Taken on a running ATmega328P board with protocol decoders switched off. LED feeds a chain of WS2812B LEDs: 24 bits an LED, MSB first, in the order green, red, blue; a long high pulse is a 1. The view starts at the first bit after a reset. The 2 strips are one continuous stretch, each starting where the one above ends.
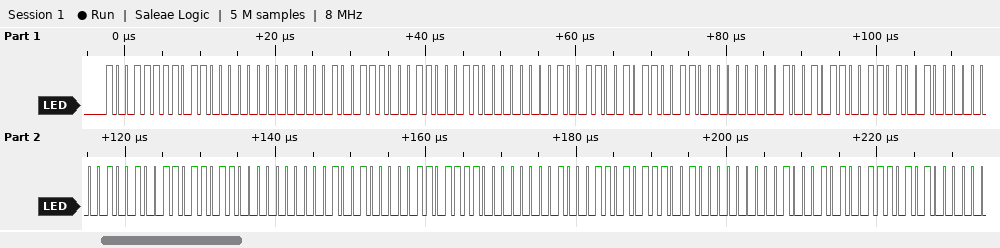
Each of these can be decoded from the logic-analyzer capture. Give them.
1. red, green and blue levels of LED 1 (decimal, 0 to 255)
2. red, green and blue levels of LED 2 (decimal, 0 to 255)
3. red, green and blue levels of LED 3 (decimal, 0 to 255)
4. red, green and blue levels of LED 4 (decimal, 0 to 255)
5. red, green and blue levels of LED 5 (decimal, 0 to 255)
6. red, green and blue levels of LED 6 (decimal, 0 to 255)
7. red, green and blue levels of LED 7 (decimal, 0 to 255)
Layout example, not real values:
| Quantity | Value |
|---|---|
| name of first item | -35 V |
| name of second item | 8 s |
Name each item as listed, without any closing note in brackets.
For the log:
| Quantity | Value |
|---|---|
| red, green and blue levels of LED 1 | 96, 159, 0 |
| red, green and blue levels of LED 2 | 99, 156, 0 |
| red, green and blue levels of LED 3 | 102, 153, 0 |
| red, green and blue levels of LED 4 | 105, 150, 0 |
| red, green and blue levels of LED 5 | 108, 147, 0 |
| red, green and blue levels of LED 6 | 111, 144, 0 |
| red, green and blue levels of LED 7 | 114, 141, 0 |
